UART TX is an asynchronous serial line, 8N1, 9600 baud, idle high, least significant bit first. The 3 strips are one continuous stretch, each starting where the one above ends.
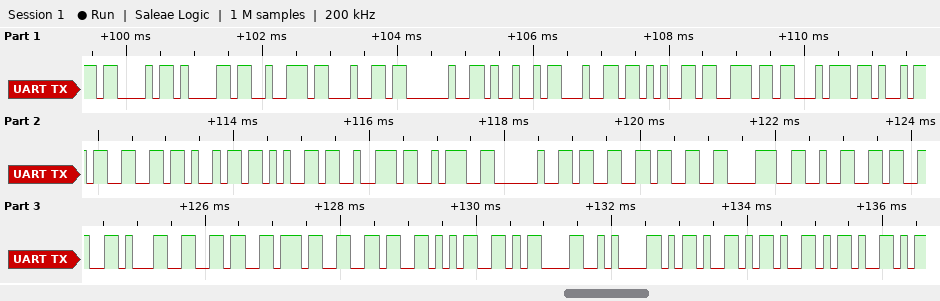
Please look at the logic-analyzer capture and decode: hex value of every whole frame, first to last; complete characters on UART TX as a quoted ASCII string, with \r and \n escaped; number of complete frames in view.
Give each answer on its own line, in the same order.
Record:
43 61 72 64 20 49 64 65 6E 74 69 66 69 65 72 3A 20 33 33 38 32 33 31 36 37 36 35 0D 0A 2D 2D 2D
"Card Identifier: 3382316765\r\n---"
32
